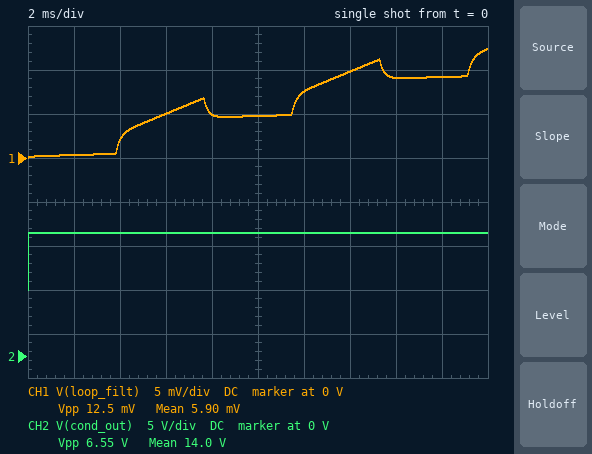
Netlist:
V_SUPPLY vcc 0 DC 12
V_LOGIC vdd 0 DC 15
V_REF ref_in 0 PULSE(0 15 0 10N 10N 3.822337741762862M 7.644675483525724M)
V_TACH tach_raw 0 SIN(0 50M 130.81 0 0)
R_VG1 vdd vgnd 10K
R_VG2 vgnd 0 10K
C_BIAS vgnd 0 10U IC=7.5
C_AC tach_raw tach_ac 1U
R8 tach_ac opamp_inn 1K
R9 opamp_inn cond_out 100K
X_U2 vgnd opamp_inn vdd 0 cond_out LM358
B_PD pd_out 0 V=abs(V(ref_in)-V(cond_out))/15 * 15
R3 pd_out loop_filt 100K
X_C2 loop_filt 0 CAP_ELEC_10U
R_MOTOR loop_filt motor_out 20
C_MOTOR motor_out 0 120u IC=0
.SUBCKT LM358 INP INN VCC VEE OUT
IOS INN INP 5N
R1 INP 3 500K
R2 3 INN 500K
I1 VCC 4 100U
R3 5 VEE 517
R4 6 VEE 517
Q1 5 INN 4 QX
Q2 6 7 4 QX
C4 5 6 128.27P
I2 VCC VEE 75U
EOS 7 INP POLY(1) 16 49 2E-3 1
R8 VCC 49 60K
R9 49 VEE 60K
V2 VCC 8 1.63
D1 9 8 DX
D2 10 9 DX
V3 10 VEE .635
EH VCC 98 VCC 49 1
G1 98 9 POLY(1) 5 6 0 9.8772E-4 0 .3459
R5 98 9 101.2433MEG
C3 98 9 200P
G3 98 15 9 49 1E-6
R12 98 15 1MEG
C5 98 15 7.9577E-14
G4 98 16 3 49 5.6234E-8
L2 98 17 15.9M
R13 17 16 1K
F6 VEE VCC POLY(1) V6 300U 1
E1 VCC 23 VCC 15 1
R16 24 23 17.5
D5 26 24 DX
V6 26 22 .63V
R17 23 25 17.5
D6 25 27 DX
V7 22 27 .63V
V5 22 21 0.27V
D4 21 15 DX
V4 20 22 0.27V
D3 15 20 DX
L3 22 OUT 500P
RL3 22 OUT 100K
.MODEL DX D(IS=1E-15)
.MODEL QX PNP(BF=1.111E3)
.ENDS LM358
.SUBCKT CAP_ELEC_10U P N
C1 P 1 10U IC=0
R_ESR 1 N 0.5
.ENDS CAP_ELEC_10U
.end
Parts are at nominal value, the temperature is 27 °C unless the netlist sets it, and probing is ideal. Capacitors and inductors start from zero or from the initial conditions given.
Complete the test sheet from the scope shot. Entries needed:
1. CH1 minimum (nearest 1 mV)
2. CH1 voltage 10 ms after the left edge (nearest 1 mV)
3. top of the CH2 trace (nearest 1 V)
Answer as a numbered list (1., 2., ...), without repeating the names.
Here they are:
1. 0 V
2. 5 mV
3. 14 V
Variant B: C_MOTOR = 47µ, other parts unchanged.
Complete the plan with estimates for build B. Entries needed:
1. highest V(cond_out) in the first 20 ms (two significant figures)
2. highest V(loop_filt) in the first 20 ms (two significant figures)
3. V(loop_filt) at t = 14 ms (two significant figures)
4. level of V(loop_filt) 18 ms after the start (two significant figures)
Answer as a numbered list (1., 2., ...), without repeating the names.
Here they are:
1. 14 V
2. 25 mV
3. 19 mV
4. 21 mV
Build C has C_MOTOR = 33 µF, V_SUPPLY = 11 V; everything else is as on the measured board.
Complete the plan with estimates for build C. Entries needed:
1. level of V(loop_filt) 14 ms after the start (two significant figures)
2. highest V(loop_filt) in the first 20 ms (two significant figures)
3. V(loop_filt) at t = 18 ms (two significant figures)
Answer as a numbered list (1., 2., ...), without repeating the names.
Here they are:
1. 24 mV
2. 32 mV
3. 27 mV
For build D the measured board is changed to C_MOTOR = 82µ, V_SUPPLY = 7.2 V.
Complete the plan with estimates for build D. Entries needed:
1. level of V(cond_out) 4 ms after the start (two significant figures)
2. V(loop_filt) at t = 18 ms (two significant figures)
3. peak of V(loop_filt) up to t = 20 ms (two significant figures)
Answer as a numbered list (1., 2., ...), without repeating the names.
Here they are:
1. 14 V
2. 13 mV
3. 16 mV
